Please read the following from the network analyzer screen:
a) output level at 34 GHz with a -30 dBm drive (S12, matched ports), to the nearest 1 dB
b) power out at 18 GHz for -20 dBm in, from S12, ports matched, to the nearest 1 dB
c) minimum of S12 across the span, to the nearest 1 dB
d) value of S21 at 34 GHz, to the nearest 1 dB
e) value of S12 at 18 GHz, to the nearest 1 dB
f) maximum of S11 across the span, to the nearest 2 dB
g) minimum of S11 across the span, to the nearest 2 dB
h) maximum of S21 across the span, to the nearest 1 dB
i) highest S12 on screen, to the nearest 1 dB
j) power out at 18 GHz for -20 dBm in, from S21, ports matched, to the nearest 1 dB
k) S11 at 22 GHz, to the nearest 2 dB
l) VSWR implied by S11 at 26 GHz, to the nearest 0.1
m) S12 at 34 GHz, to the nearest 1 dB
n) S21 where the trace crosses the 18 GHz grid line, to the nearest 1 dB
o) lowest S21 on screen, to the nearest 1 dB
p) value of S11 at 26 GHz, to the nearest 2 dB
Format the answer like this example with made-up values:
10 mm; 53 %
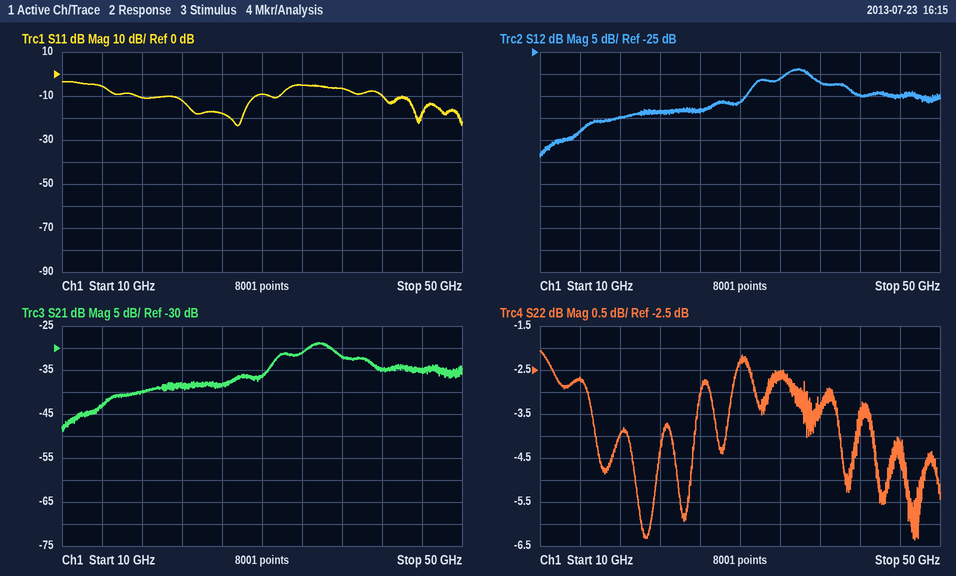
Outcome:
-61 dBm; -60 dBm; -49 dB; -31 dB; -40 dB; -4 dB; -24 dB; -29 dB; -29 dB; -60 dBm; -12 dB; 1.3; -31 dB; -40 dB; -49 dB; -18 dB
